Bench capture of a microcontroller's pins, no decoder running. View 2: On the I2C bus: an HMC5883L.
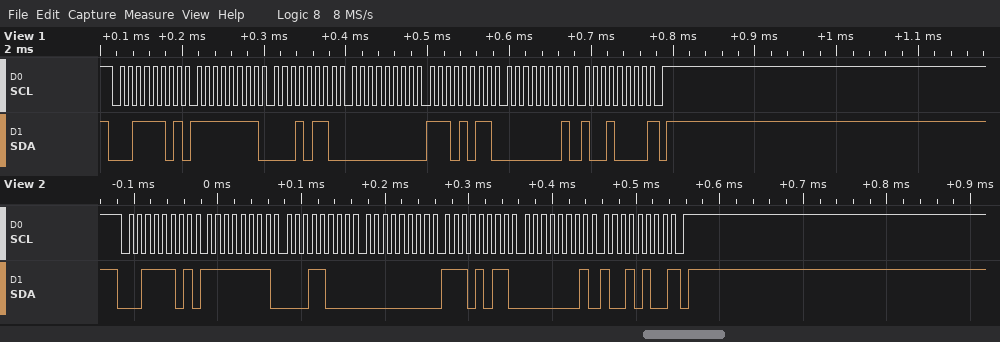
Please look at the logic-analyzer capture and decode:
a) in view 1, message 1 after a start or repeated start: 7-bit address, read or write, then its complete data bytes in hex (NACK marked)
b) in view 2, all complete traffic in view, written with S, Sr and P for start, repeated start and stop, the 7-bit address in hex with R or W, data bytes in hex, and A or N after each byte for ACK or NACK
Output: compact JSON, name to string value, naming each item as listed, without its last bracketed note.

{"in view 1, message 1 after a start or repeated start: 7-bit address, read or write, then its complete data bytes in hex": "0x1E read: FF 16 00 EB 01 90 NACK", "in view 2, all complete traffic in view, written with S, Sr and P for start, repeated start and stop, the 7-bit address in hex with R or W, data bytes in hex, and A or N after each byte for ACK or NACK": "S 1ER A FF A 18 A 00 A EB A 01 A 94 N P"}
